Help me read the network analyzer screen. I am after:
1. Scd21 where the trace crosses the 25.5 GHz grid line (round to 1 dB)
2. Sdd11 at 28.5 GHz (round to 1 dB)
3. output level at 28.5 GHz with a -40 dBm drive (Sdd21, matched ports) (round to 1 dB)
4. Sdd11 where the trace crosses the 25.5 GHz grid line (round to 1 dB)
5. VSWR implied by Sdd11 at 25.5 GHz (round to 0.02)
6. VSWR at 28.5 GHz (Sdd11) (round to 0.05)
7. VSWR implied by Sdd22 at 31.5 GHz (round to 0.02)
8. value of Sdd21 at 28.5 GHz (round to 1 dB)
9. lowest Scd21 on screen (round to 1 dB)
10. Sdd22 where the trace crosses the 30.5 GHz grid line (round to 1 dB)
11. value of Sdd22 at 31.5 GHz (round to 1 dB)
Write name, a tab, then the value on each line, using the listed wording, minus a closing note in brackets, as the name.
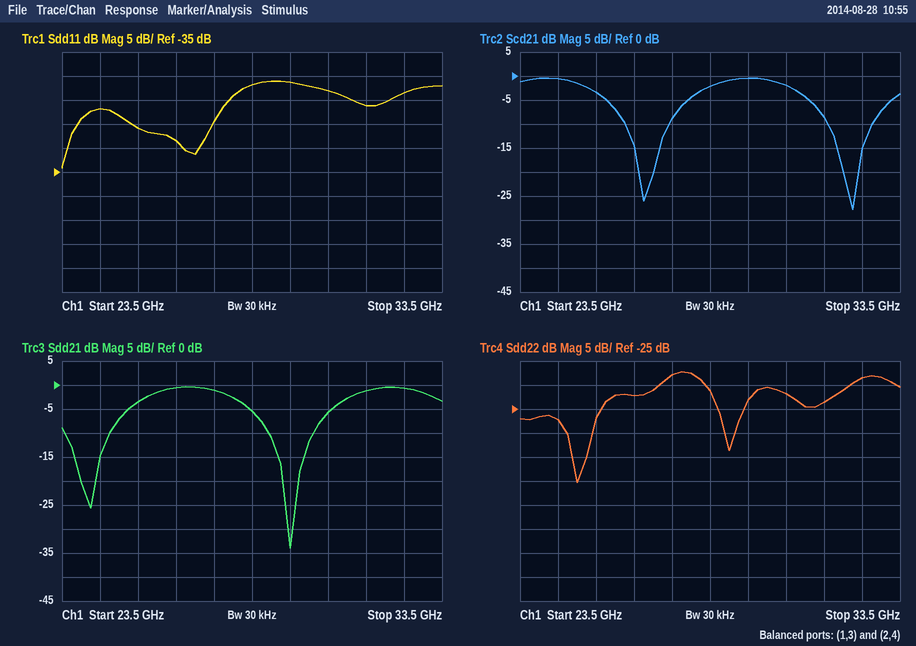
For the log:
Scd21 where the trace crosses the 25.5 GHz grid line	-3 dB
Sdd11 at 28.5 GHz	-17 dB
output level at 28.5 GHz with a -40 dBm drive (Sdd21, matched ports)	-45 dBm
Sdd11 where the trace crosses the 25.5 GHz grid line	-26 dB
VSWR implied by Sdd11 at 25.5 GHz	1.10
VSWR at 28.5 GHz (Sdd11)	1.35
VSWR implied by Sdd22 at 31.5 GHz	1.14
value of Sdd21 at 28.5 GHz	-5 dB
lowest Scd21 on screen	-28 dB
Sdd22 where the trace crosses the 30.5 GHz grid line	-22 dB
value of Sdd22 at 31.5 GHz	-24 dB
